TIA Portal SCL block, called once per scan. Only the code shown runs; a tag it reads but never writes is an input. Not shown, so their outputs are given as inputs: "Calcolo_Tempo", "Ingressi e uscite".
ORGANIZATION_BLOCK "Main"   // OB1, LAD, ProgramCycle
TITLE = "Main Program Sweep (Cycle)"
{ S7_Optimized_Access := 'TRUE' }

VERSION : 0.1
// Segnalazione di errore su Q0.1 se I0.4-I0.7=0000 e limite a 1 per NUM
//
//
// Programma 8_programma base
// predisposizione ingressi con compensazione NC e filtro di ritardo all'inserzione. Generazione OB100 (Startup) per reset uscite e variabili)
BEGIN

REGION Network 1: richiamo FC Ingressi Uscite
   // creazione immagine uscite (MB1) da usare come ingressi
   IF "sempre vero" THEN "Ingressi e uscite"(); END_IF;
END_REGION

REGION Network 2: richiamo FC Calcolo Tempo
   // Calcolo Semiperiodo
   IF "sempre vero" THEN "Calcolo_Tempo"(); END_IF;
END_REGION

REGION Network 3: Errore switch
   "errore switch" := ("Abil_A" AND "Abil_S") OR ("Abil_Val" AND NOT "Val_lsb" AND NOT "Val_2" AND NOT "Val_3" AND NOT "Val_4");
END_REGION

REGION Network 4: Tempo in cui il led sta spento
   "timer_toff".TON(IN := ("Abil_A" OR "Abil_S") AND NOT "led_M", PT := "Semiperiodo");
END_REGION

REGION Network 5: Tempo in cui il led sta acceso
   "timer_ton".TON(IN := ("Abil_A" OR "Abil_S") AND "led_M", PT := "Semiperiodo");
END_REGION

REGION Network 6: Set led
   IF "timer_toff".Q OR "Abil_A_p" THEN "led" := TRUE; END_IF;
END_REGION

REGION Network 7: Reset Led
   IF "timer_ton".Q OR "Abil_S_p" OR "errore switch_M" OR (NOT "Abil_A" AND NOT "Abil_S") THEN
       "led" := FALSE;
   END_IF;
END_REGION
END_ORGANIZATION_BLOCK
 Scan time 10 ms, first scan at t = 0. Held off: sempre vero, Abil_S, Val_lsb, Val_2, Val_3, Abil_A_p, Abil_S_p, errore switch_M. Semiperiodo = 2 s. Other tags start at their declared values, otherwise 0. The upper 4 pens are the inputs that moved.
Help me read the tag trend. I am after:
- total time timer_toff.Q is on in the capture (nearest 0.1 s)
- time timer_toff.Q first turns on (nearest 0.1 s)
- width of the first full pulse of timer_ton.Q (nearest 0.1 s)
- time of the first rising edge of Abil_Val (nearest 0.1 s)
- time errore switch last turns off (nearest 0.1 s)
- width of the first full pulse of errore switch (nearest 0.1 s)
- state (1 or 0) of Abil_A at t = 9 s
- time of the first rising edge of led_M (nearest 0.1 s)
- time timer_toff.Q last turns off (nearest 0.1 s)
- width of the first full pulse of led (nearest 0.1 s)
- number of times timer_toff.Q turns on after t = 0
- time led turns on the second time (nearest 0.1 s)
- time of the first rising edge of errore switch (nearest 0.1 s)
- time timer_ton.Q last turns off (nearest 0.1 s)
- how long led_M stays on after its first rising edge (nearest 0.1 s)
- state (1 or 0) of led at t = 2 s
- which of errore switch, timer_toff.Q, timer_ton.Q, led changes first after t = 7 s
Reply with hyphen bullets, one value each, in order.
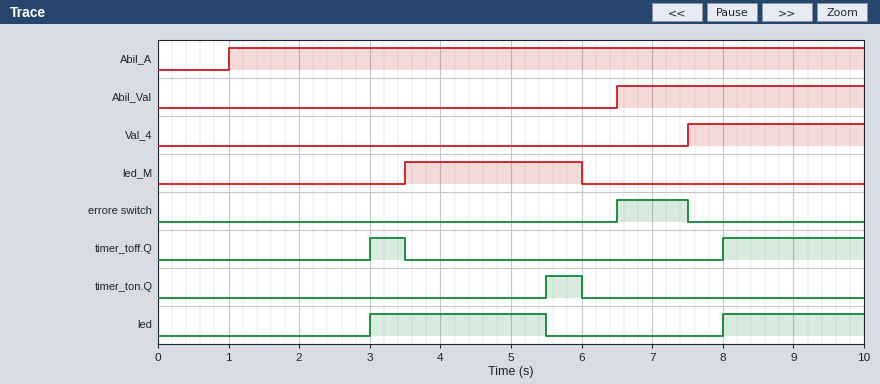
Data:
- 2.5 s
- 3.0 s
- 0.5 s
- 6.5 s
- 7.5 s
- 1.0 s
- 1
- 3.5 s
- 3.5 s
- 2.5 s
- 2
- 8.0 s
- 6.5 s
- 6.0 s
- 2.5 s
- 0
- errore switch
